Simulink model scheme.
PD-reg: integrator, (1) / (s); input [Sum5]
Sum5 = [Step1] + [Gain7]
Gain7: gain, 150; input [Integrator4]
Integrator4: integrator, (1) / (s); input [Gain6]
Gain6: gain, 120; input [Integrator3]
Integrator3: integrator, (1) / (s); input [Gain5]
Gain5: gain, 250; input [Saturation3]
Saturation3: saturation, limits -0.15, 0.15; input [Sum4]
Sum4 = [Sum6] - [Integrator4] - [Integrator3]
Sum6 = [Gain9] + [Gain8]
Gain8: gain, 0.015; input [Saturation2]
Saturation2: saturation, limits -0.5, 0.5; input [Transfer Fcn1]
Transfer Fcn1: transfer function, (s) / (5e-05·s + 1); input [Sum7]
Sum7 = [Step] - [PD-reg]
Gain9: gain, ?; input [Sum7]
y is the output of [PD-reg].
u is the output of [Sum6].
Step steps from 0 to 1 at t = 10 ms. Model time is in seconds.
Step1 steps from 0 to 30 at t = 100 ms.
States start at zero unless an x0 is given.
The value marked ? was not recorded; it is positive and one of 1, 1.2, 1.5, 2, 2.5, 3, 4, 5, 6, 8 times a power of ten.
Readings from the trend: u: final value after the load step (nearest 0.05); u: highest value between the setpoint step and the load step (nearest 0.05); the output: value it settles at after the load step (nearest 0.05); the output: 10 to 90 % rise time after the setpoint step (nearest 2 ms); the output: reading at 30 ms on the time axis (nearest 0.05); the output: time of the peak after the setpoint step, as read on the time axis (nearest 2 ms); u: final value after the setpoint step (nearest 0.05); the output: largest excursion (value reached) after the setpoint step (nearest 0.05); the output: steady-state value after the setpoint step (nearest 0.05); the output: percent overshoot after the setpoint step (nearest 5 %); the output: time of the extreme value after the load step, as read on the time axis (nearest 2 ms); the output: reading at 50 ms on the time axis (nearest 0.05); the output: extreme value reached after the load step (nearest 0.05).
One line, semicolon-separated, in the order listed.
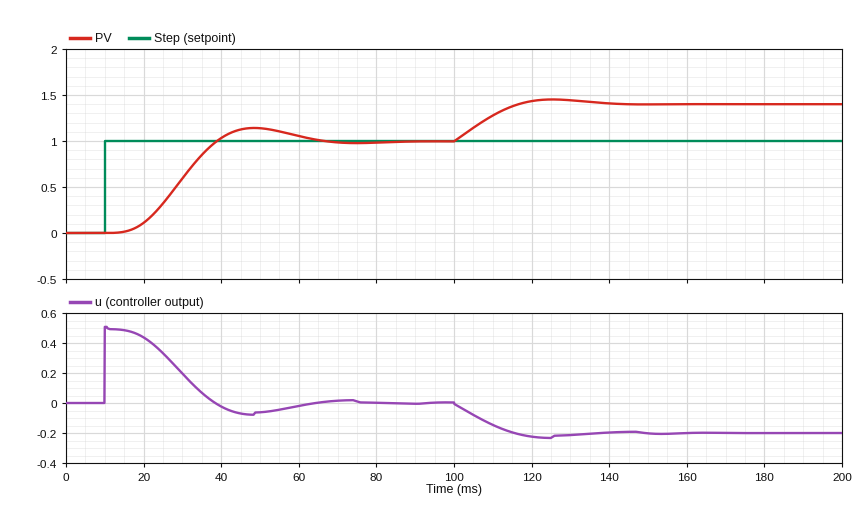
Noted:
-0.20; 0.50; 1.40; 16 ms; 0.60; 48 ms; 0.00; 1.15; 1.00; 15 %; 126 ms; 1.15; 1.45
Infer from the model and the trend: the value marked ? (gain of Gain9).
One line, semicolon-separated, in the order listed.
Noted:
0.5
